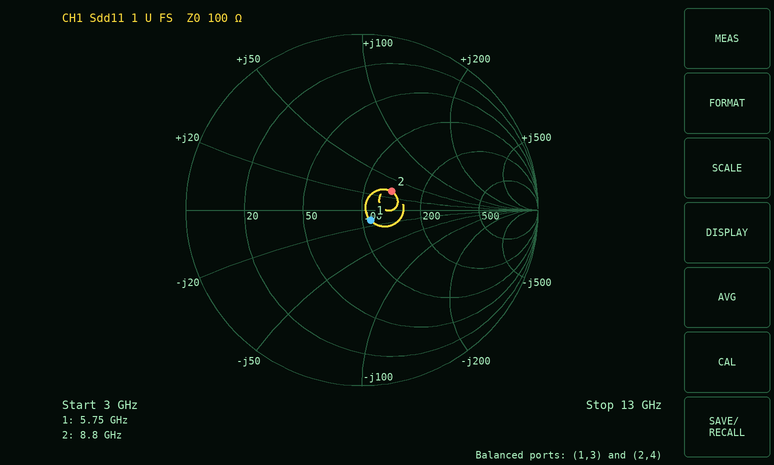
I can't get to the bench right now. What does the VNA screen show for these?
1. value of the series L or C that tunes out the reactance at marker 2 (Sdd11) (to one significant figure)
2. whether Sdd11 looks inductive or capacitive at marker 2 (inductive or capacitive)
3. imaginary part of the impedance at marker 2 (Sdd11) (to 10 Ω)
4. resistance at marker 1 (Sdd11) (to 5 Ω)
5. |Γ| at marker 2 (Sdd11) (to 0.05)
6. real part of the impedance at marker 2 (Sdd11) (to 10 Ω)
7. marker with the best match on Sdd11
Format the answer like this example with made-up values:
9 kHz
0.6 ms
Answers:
600 fF
inductive
+30 Ω
110 Ω
0.20
140 Ω
marker 1
